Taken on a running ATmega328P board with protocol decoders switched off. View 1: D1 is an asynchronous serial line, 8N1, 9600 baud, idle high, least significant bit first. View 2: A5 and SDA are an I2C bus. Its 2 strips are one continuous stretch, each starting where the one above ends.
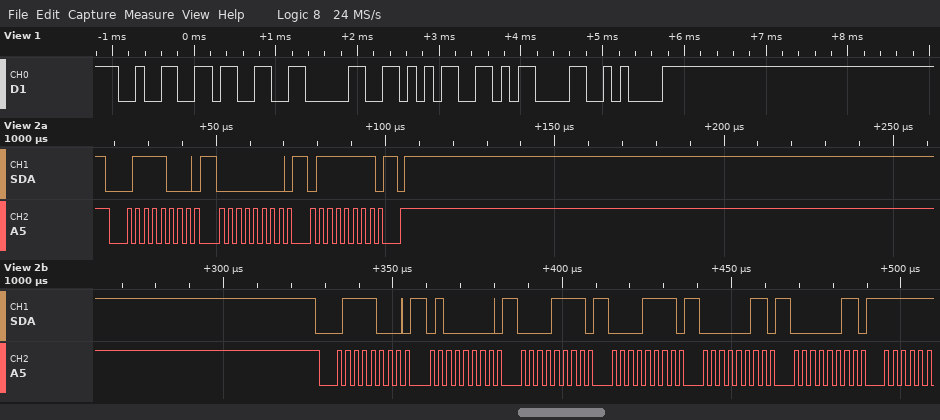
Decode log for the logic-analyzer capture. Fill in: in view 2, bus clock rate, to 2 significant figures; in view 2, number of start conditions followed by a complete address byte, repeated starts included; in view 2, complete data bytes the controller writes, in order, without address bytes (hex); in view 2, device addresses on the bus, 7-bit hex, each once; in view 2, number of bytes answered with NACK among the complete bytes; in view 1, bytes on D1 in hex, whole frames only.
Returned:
400 kHz
2
00 7F 40 0F 0F 03 03
0x3C
0
32 33 30 35 0D 0A
